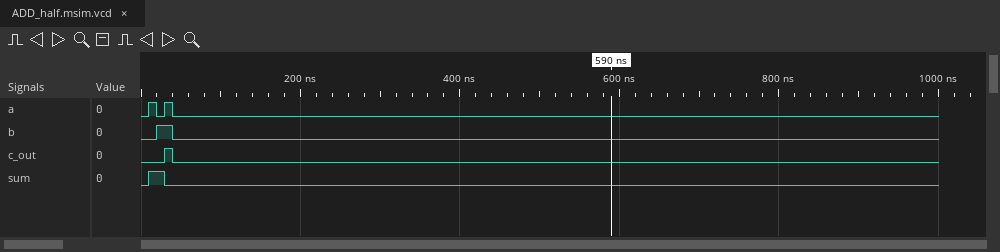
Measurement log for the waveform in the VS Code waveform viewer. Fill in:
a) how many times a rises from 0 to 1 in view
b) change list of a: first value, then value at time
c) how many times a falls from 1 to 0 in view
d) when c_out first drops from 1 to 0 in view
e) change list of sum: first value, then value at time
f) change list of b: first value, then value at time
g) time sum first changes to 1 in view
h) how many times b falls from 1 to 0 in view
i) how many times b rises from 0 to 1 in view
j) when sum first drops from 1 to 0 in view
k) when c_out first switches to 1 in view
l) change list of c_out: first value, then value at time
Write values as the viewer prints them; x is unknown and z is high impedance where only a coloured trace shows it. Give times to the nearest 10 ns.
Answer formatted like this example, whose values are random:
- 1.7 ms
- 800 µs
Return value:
- 2
- 0, 1 at 10 ns, 0 at 20 ns, 1 at 30 ns, 0 at 40 ns
- 2
- 40 ns
- 0, 1 at 10 ns, 0 at 30 ns
- 0, 1 at 20 ns, 0 at 40 ns
- 10 ns
- 1
- 1
- 30 ns
- 30 ns
- 0, 1 at 30 ns, 0 at 40 ns
